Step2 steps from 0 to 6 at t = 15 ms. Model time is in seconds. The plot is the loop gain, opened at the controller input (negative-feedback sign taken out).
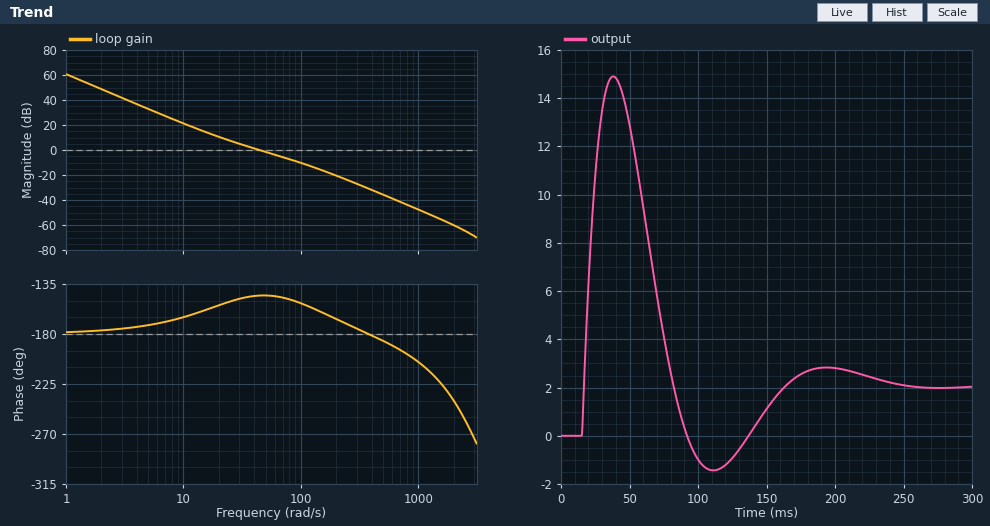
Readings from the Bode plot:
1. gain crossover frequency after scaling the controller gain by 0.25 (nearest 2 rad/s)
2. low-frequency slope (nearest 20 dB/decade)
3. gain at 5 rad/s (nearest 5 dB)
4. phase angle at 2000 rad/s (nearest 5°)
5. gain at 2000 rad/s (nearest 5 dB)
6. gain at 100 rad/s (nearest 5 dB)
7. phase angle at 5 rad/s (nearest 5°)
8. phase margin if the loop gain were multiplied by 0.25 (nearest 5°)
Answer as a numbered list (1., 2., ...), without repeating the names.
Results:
1. 18 rad/s
2. -40 dB/decade
3. 35 dB
4. -240°
5. -60 dB
6. -10 dB
7. -170°
8. 25°
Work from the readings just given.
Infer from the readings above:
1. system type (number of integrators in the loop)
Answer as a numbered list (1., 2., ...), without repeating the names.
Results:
1. 2
